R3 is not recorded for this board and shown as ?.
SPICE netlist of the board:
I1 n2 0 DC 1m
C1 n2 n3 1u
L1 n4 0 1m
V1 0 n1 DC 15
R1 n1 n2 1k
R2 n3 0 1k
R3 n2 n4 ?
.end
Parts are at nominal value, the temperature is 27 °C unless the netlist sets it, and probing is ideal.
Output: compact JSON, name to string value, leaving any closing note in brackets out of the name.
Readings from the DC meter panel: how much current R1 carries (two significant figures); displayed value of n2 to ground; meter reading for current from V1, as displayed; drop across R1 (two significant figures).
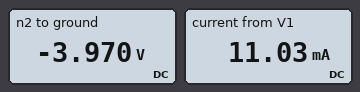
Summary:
{"how much current R1 carries": "11 mA", "displayed value of n2 to ground": "-3.970 V", "meter reading for current from V1, as displayed": "11.03 mA", "drop across R1": "11 V"}
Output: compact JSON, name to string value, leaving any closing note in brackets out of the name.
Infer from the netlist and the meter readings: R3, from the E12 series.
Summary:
{"R3, from the E12 series": "330 Ω"}
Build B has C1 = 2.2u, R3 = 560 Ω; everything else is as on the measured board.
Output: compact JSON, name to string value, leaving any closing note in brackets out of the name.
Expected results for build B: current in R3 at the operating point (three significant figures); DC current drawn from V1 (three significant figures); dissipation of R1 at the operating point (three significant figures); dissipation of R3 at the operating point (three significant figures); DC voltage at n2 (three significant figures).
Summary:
{"current in R3 at the operating point": "10.3 mA", "DC current drawn from V1": "9.26 mA", "dissipation of R1 at the operating point": "85.7 mW", "dissipation of R3 at the operating point": "58.9 mW", "DC voltage at n2": "-5.74 V"}
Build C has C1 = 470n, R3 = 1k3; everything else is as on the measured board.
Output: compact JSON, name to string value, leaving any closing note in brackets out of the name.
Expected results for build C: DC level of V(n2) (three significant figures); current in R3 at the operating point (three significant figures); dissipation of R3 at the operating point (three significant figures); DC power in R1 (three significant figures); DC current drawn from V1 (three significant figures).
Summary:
{"DC level of V(n2)": "-9.04 V", "current in R3 at the operating point": "6.96 mA", "dissipation of R3 at the operating point": "62.9 mW", "DC power in R1": "35.5 mW", "DC current drawn from V1": "5.96 mA"}
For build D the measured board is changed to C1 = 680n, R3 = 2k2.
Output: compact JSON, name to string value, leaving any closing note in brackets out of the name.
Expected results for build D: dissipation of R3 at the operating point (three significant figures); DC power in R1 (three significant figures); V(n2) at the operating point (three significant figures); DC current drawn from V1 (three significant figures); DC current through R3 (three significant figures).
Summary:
{"dissipation of R3 at the operating point": "55.0 mW", "DC power in R1": "16.0 mW", "V(n2) at the operating point": "-11.0 V", "DC current drawn from V1": "4.00 mA", "DC current through R3": "5.00 mA"}
